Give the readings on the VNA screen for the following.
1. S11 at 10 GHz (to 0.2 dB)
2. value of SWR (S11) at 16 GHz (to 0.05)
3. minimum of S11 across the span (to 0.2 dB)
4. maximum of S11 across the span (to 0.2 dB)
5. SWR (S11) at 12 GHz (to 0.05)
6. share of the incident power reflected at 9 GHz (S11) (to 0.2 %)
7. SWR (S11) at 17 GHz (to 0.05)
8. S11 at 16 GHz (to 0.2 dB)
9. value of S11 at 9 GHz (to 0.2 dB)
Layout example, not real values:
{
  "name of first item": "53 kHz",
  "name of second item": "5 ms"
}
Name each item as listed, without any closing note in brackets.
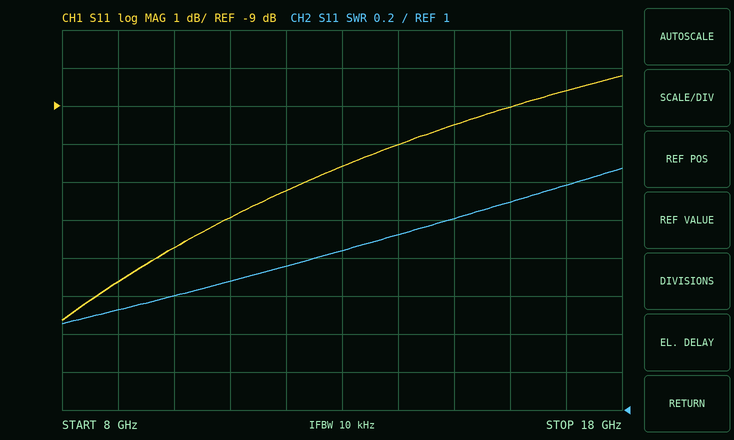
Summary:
{
  "S11 at 10 GHz": "-12.8 dB",
  "value of SWR (S11) at 16 GHz": "2.10",
  "minimum of S11 across the span": "-14.6 dB",
  "maximum of S11 across the span": "-8.2 dB",
  "SWR (S11) at 12 GHz": "1.75",
  "share of the incident power reflected at 9 GHz (S11)": "4.4 %",
  "SWR (S11) at 17 GHz": "2.20",
  "S11 at 16 GHz": "-9.0 dB",
  "value of S11 at 9 GHz": "-13.6 dB"
}
